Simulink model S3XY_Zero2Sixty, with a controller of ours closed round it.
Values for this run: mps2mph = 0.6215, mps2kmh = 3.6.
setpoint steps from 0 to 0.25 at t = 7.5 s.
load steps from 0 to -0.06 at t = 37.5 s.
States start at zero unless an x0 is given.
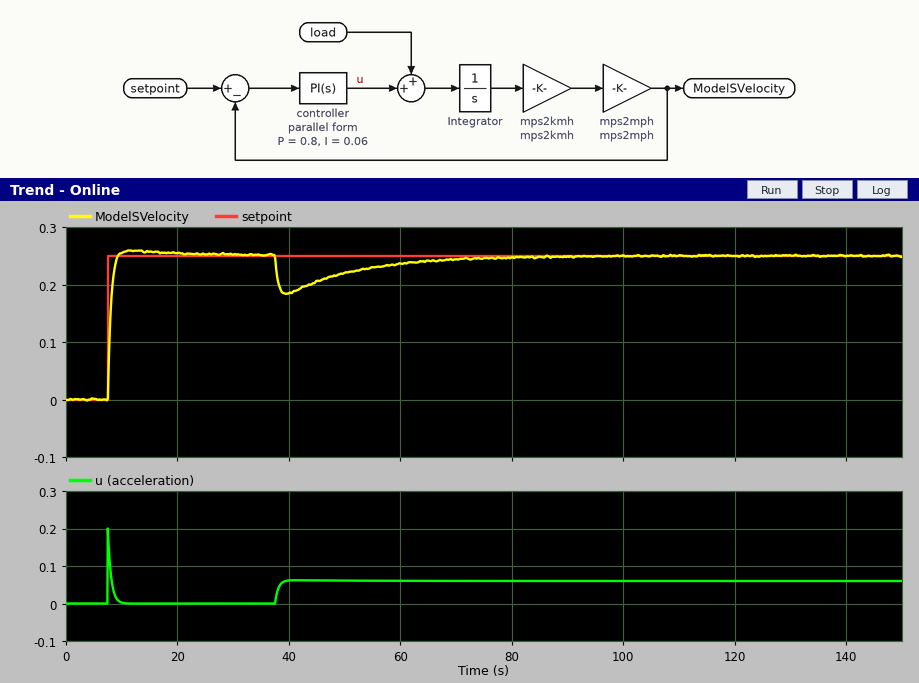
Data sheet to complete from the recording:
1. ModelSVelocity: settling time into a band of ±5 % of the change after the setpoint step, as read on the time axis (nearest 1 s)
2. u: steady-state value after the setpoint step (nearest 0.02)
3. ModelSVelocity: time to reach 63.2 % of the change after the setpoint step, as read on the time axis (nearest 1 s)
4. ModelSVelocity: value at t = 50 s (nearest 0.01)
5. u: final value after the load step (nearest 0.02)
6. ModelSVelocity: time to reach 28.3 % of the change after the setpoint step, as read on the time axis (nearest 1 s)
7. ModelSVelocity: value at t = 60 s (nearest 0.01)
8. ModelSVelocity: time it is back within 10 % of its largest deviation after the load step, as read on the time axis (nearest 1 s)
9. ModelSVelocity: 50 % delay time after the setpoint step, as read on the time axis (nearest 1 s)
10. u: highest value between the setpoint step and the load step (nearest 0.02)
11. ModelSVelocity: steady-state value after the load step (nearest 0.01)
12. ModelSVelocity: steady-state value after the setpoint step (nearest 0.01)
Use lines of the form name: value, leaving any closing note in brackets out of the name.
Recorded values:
ModelSVelocity: settling time into a band of ±5 % of the change after the setpoint step, as read on the time axis: 9 s
u: steady-state value after the setpoint step: 0.00
ModelSVelocity: time to reach 63.2 % of the change after the setpoint step, as read on the time axis: 8 s
ModelSVelocity: value at t = 50 s: 0.22
u: final value after the load step: 0.06
ModelSVelocity: time to reach 28.3 % of the change after the setpoint step, as read on the time axis: 8 s
ModelSVelocity: value at t = 60 s: 0.24
ModelSVelocity: time it is back within 10 % of its largest deviation after the load step, as read on the time axis: 69 s
ModelSVelocity: 50 % delay time after the setpoint step, as read on the time axis: 8 s
u: highest value between the setpoint step and the load step: 0.20
ModelSVelocity: steady-state value after the load step: 0.25
ModelSVelocity: steady-state value after the setpoint step: 0.25
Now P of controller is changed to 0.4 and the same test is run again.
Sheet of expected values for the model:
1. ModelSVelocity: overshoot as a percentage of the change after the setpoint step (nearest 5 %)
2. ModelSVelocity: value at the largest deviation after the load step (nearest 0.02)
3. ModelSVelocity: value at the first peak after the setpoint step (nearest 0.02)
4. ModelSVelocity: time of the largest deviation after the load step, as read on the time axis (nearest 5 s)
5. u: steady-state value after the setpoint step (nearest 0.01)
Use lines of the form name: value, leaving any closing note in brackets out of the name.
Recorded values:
ModelSVelocity: overshoot as a percentage of the change after the setpoint step: 10 %
ModelSVelocity: value at the largest deviation after the load step: 0.14
ModelSVelocity: value at the first peak after the setpoint step: 0.28
ModelSVelocity: time of the largest deviation after the load step, as read on the time axis: 40 s
u: steady-state value after the setpoint step: 0.00
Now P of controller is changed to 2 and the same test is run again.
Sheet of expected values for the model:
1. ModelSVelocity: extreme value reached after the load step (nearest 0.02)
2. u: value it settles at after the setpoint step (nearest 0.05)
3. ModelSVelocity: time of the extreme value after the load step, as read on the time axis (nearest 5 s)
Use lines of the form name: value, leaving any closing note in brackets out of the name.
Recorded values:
ModelSVelocity: extreme value reached after the load step: 0.22
u: value it settles at after the setpoint step: 0.00
ModelSVelocity: time of the extreme value after the load step, as read on the time axis: 40 s
